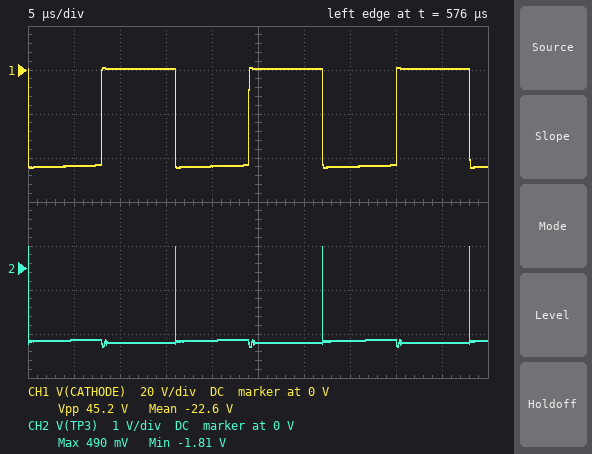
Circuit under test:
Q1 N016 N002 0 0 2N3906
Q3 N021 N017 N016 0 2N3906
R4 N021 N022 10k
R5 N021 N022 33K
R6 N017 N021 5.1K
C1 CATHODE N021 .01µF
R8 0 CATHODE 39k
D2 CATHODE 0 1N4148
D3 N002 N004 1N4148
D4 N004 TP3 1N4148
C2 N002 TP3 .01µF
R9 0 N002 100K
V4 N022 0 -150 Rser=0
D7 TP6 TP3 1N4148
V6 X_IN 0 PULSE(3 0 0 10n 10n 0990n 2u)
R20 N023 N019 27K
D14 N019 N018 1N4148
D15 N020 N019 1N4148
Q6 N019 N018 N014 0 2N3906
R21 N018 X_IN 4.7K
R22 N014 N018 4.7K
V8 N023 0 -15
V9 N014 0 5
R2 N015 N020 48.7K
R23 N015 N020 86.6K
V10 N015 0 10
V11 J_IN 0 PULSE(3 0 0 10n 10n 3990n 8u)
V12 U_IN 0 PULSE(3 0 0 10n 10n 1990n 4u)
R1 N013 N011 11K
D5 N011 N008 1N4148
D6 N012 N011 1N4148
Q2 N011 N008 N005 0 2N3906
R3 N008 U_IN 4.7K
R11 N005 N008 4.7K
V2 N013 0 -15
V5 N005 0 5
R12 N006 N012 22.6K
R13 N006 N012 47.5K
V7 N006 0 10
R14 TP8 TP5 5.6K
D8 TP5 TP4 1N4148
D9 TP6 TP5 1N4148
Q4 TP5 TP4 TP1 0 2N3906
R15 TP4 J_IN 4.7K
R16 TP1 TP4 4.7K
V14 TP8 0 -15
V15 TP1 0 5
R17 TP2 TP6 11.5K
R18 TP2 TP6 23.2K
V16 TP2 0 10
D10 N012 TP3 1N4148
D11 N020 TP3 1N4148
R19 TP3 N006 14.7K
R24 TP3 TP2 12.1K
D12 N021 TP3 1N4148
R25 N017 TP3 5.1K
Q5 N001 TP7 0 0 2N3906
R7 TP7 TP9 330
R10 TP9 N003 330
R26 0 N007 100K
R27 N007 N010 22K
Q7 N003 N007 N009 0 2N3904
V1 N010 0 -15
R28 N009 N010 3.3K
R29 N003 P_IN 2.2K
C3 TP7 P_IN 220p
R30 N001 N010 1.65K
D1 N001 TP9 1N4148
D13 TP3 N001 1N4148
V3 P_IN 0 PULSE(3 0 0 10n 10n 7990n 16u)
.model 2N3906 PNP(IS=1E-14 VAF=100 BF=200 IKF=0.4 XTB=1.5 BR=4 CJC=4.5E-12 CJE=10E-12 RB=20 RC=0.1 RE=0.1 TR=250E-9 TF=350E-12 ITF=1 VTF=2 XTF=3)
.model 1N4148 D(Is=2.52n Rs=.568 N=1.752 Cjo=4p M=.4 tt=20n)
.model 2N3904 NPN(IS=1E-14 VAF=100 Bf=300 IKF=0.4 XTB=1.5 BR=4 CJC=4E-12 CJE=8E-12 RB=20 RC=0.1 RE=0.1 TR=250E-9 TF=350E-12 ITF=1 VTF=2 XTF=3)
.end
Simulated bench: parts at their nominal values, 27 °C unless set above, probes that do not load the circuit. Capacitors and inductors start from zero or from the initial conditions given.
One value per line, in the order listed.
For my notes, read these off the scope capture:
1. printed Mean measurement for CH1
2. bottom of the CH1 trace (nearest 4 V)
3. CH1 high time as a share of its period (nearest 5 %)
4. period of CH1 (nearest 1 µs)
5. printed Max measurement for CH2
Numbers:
-22.6 V
-44 V
50 %
16 µs
490 mV
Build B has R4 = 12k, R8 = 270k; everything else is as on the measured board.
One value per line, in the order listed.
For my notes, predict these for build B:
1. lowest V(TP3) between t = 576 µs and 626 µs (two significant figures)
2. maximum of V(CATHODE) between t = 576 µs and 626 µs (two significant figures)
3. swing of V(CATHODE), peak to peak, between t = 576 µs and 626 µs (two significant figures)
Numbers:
-1.7 V
650 mV
45 V
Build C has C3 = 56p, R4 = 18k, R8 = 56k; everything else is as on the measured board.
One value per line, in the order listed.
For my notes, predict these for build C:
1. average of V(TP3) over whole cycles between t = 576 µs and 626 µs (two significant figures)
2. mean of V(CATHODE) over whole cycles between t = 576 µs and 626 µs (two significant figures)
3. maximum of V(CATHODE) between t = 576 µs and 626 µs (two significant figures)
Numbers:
-1.6 V
-21 V
740 mV
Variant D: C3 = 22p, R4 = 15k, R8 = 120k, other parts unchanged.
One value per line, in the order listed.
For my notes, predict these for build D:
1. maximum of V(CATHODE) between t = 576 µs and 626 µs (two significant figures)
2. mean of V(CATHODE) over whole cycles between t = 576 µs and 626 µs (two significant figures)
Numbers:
700 mV
-21 V
